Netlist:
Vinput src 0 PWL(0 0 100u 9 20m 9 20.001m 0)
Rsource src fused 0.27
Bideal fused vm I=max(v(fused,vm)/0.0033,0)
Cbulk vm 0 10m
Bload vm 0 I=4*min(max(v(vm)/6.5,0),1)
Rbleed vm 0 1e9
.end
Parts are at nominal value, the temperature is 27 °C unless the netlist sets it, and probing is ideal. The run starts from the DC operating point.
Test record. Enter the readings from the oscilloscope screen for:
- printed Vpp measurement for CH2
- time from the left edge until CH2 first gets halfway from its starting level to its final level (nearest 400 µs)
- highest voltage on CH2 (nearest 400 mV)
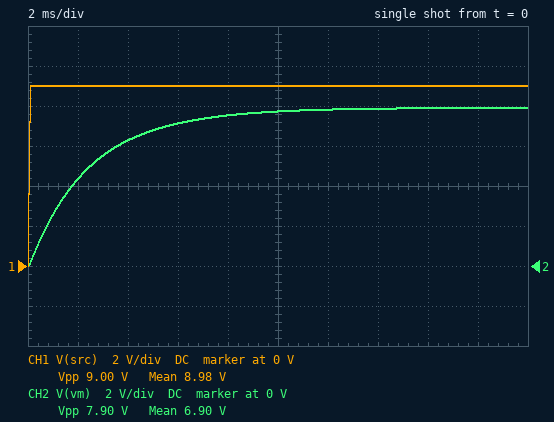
7.90 V
1.6 ms
8.0 V
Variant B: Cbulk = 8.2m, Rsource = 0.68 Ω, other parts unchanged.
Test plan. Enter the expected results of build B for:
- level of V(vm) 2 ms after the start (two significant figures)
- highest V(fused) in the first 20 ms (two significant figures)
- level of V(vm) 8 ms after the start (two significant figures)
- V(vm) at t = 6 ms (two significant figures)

2.5 V
6.3 V
5.5 V
4.9 V
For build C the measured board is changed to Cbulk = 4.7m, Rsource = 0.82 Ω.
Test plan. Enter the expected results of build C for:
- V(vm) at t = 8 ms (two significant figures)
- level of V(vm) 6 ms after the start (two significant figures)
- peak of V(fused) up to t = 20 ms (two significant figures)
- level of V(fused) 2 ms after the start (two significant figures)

5.7 V
5.4 V
6.0 V
3.2 V
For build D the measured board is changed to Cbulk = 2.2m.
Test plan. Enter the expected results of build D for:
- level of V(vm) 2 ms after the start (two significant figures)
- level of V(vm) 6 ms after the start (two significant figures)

7.6 V
7.9 V
